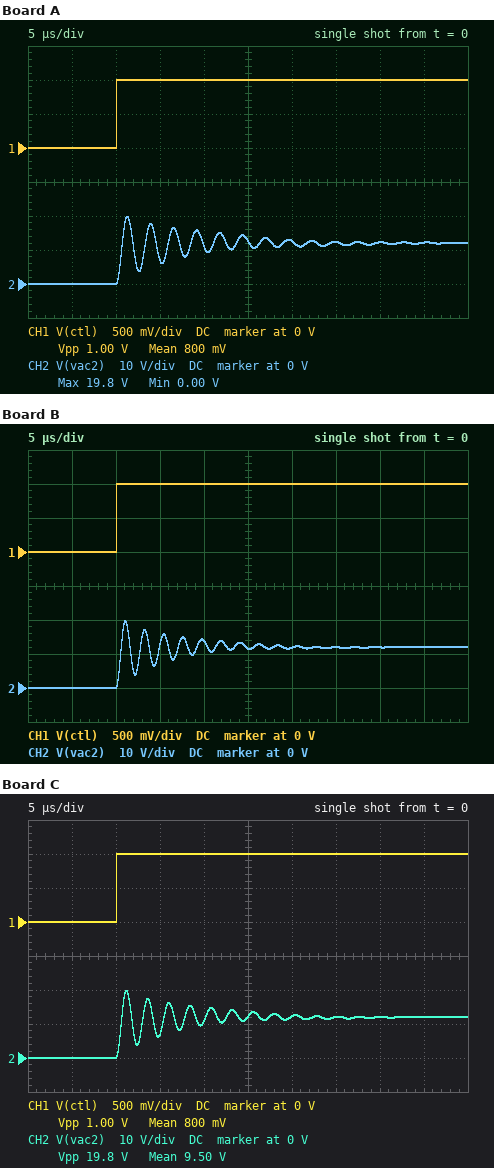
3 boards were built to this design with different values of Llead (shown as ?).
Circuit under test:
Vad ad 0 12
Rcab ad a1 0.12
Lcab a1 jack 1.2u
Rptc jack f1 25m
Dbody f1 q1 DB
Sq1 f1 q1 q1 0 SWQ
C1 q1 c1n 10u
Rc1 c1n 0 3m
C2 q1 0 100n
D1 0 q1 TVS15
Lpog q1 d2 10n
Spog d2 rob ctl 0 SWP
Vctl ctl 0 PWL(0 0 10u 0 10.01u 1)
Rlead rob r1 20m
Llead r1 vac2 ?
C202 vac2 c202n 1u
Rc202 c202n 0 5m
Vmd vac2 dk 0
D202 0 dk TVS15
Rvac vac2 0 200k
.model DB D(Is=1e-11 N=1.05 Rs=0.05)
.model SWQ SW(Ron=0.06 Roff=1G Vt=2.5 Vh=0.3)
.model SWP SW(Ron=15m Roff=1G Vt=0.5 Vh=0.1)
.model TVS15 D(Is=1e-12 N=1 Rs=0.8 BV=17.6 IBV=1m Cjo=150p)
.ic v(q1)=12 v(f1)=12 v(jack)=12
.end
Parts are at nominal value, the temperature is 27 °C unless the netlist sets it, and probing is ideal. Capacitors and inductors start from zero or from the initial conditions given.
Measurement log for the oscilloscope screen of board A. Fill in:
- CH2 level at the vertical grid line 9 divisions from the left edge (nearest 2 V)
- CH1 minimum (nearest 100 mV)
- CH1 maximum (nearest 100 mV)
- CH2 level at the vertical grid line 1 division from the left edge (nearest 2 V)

12 V
0 V
1.0 V
0 V
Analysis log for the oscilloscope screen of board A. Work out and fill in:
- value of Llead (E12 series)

180 nH
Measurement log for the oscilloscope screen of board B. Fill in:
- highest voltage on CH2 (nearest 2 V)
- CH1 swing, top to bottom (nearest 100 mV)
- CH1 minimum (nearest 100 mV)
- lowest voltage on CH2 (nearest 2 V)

20 V
1.0 V
0 V
0 V
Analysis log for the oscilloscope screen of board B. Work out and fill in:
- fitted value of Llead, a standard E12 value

120 nH
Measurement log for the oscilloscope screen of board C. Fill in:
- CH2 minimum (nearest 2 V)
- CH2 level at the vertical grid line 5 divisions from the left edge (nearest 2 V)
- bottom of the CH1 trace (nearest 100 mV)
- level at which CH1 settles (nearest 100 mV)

0 V
12 V
0 V
1.0 V
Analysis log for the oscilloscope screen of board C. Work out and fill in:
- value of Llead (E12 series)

150 nH
